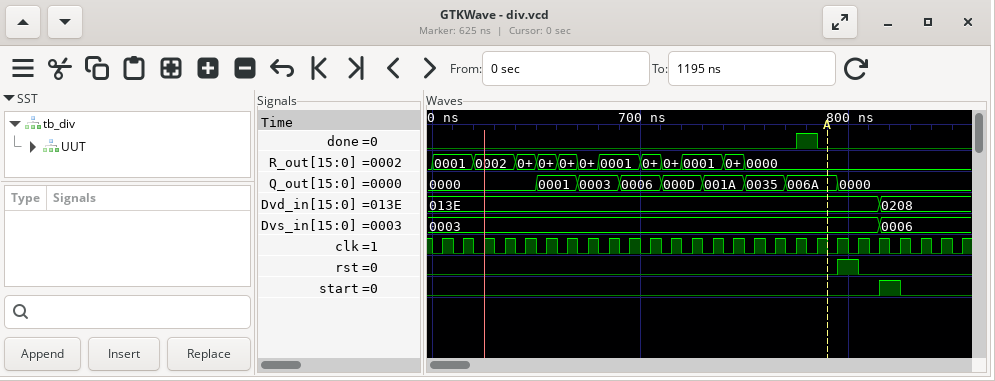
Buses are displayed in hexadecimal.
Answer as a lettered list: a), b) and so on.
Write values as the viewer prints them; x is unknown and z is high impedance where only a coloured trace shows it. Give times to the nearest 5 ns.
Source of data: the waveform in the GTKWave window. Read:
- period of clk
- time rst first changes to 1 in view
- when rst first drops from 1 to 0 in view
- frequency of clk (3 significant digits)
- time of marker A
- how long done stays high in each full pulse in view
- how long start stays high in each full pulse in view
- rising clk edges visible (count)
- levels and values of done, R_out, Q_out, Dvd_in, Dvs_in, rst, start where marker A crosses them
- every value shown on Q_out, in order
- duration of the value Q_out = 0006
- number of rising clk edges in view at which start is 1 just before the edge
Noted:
a) 10 ns
b) 795 ns
c) 805 ns
d) 100 MHz
e) 790 ns
f) 10 ns
g) 10 ns
h) 26
i) done=0, R_out=0000, Q_out=006A, Dvd_in=013E, Dvs_in=0003, rst=0, start=0
j) 0000, 0001, 0003, 0006, 000D, 001A, 0035, 006A, 0000
k) 20 ns
l) 1
